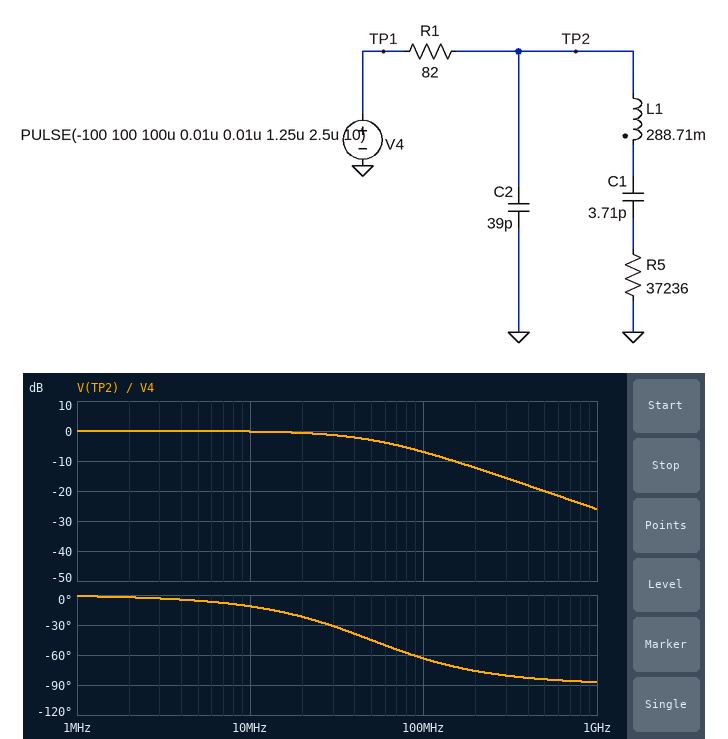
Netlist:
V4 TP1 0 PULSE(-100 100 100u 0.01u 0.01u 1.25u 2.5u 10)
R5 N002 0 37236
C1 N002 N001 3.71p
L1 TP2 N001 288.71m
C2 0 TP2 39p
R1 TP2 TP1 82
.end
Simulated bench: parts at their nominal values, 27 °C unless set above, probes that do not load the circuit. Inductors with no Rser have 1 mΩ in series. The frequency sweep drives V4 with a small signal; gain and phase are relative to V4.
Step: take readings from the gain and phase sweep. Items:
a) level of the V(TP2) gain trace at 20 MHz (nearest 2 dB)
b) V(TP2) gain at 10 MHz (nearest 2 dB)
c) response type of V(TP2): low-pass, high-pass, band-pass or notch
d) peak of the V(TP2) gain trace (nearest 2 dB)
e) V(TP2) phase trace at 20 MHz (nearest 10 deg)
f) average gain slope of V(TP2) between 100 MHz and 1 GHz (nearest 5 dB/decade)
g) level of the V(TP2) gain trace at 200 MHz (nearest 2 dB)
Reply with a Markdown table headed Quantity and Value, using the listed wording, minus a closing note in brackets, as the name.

| Quantity | Value |
|---|---|
| level of the V(TP2) gain trace at 20 MHz | 0 dB |
| V(TP2) gain at 10 MHz | 0 dB |
| response type of V(TP2): low-pass, high-pass, band-pass or notch | low-pass |
| peak of the V(TP2) gain trace | 0 dB |
| V(TP2) phase trace at 20 MHz | -20 deg |
| average gain slope of V(TP2) between 100 MHz and 1 GHz | -20 dB/decade |
| level of the V(TP2) gain trace at 200 MHz | -12 dB |
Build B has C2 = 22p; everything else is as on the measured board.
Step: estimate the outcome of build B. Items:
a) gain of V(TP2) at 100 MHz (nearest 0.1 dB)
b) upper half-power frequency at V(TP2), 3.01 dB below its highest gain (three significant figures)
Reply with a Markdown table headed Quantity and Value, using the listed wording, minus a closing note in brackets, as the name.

| Quantity | Value |
|---|---|
| gain of V(TP2) at 100 MHz | -3.6 dB |
| upper half-power frequency at V(TP2), 3.01 dB below its highest gain | 88.2 MHz |
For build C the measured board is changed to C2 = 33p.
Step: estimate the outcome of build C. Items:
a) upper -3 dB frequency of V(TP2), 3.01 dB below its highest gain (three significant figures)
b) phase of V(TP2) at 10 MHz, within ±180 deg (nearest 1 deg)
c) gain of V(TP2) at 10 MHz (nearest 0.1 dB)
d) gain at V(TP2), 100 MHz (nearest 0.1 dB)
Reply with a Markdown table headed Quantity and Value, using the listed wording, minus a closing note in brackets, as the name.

| Quantity | Value |
|---|---|
| upper -3 dB frequency of V(TP2), 3.01 dB below its highest gain | 58.8 MHz |
| phase of V(TP2) at 10 MHz, within ±180 deg | -10 deg |
| gain of V(TP2) at 10 MHz | -0.1 dB |
| gain at V(TP2), 100 MHz | -5.9 dB |
